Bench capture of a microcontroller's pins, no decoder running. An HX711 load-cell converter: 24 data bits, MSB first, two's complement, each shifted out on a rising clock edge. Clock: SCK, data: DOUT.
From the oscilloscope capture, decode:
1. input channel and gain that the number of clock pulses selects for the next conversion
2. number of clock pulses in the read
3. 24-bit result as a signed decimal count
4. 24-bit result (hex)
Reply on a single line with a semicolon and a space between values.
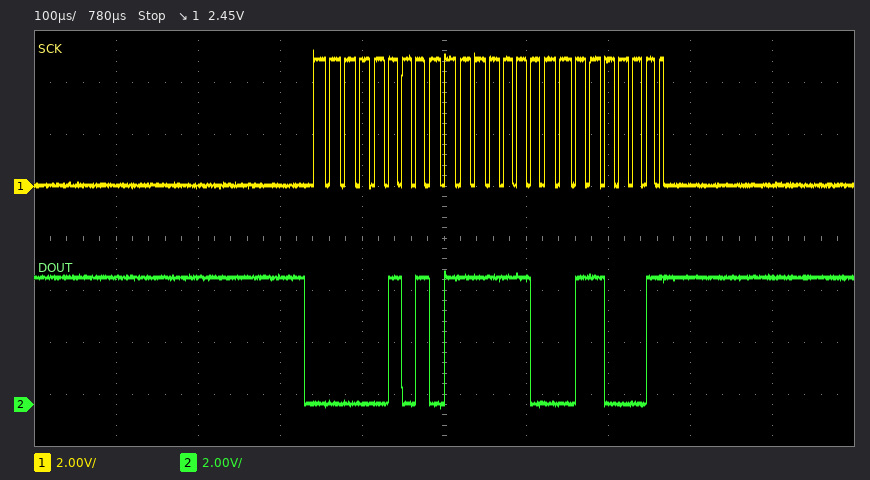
channel A, gain 128; 25; 359985; 0x057E31
